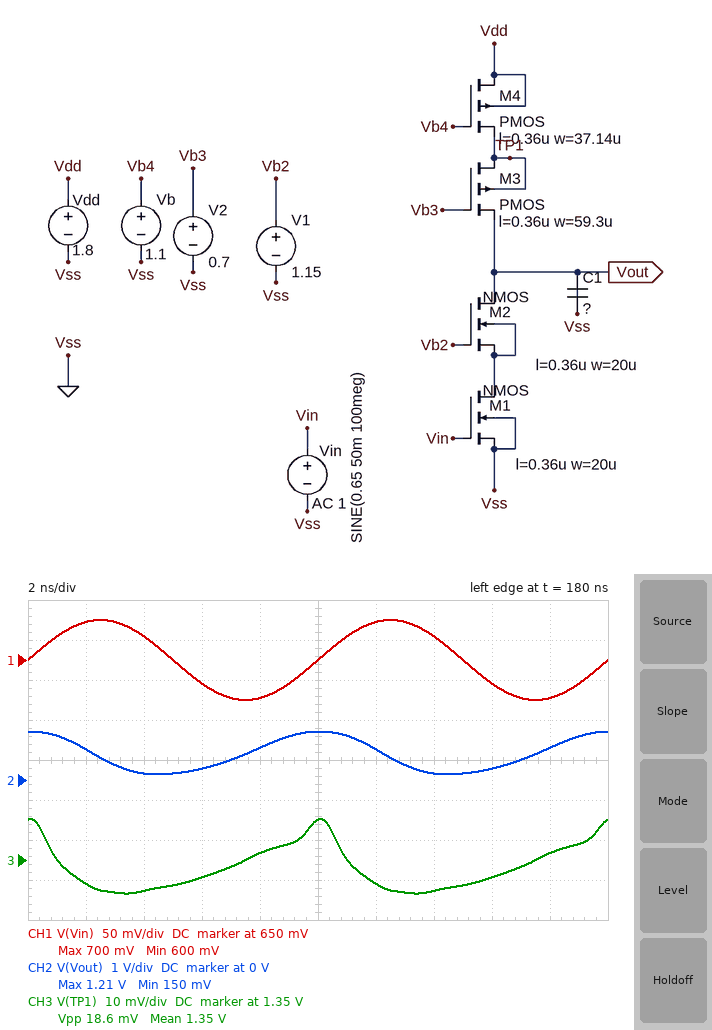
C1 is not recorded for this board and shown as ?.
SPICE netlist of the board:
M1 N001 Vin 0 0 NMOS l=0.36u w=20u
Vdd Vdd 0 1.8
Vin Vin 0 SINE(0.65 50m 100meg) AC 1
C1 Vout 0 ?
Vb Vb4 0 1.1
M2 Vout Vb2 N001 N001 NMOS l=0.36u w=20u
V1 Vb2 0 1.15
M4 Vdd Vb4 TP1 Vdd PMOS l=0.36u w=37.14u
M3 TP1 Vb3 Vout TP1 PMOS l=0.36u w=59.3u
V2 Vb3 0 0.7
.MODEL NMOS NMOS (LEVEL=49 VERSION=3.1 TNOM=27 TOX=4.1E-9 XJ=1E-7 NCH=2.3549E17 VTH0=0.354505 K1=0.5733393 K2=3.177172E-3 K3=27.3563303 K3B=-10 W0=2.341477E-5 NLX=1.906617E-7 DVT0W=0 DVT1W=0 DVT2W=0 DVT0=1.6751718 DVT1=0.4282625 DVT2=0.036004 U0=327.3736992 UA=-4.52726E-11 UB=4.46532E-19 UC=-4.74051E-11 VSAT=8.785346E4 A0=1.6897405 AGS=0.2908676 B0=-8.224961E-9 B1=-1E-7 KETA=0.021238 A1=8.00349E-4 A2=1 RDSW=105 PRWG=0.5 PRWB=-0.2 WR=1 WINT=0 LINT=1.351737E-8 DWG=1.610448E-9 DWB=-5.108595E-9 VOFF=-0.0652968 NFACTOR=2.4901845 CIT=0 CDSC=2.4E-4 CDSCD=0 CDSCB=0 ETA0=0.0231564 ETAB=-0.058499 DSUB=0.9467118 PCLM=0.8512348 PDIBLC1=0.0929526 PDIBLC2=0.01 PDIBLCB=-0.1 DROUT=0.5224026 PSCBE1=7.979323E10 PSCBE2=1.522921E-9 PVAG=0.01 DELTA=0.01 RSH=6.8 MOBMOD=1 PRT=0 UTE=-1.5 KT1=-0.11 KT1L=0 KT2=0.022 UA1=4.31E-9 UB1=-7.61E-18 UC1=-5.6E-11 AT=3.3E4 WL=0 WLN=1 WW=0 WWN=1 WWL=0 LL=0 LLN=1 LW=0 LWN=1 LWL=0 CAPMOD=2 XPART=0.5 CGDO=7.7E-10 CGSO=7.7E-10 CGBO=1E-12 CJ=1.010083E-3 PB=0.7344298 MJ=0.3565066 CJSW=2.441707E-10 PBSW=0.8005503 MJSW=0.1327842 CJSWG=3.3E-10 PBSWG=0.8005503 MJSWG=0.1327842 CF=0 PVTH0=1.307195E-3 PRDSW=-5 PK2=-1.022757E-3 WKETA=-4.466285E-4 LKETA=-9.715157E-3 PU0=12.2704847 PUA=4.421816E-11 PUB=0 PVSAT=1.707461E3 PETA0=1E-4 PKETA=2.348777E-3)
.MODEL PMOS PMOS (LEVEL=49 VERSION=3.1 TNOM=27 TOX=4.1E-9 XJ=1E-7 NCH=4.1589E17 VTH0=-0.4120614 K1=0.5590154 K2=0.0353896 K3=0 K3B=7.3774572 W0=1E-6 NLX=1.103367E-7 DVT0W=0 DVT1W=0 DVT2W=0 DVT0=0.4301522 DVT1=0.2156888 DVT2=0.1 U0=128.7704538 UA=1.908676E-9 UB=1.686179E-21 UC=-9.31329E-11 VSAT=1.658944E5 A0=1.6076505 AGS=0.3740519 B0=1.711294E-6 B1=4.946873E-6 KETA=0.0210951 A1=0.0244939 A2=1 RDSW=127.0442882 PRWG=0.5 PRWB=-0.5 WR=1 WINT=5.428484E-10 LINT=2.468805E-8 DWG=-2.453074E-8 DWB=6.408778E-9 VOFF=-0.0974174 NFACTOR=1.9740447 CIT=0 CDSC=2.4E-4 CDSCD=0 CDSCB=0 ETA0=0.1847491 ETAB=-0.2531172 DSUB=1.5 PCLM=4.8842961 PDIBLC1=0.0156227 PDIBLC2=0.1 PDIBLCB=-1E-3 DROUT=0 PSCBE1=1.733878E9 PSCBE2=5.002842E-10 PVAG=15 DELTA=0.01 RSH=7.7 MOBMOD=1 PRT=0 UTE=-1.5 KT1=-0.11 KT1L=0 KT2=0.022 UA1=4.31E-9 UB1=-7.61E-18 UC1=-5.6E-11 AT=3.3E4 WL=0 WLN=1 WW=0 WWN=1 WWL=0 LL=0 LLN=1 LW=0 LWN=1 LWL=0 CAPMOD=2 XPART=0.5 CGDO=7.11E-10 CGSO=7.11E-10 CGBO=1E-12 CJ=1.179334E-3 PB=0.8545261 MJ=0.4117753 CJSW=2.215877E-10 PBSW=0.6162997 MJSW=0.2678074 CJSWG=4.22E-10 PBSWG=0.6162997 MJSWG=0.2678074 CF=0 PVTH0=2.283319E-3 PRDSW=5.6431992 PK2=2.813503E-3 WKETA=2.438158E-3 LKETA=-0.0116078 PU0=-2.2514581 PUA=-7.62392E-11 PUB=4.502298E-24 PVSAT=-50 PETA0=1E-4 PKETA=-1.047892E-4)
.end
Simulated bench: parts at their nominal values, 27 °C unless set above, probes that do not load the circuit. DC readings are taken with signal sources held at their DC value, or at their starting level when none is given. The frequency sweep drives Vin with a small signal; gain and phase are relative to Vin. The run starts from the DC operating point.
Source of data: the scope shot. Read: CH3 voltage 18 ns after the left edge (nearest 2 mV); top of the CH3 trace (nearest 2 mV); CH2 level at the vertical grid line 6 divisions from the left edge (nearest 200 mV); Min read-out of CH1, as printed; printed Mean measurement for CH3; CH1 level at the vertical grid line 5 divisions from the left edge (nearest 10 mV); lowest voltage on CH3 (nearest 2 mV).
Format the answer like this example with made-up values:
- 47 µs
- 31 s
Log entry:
- 1.352 V
- 1.360 V
- 800 mV
- 600 mV
- 1.35 V
- 650 mV
- 1.342 V
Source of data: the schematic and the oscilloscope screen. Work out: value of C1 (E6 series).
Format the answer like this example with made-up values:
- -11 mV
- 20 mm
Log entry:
- 220 fF
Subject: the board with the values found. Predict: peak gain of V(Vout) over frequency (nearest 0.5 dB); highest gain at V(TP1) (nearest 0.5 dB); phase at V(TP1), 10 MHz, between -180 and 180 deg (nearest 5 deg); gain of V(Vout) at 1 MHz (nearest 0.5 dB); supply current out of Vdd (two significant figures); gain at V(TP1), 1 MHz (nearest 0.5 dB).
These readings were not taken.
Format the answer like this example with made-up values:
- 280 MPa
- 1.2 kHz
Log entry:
- 47.0 dB
- 41.0 dB
- 110 deg
- 47.0 dB
- 190 µA
- 40.5 dB
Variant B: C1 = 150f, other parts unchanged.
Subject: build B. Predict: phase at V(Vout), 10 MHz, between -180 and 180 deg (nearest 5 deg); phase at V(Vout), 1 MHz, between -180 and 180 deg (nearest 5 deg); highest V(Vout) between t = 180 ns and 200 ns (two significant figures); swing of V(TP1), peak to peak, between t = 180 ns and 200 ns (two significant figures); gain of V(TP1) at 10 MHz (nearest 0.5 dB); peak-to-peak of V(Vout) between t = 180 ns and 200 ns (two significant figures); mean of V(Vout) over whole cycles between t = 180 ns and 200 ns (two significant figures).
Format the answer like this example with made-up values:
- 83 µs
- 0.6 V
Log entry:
- 115 deg
- 170 deg
- 1.4 V
- 130 mV
- 33.5 dB
- 1.3 V
- 760 mV
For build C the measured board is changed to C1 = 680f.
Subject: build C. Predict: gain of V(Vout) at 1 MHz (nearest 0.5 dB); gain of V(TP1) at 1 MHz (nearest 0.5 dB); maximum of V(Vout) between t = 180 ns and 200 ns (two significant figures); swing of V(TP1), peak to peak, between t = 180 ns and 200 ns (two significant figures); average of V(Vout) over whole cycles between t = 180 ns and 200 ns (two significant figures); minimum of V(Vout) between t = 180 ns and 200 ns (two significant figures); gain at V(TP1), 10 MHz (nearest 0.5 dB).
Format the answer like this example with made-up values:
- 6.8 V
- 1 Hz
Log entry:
- 46.0 dB
- 39.5 dB
- 600 mV
- 4.3 mV
- 390 mV
- 180 mV
- 26.0 dB
